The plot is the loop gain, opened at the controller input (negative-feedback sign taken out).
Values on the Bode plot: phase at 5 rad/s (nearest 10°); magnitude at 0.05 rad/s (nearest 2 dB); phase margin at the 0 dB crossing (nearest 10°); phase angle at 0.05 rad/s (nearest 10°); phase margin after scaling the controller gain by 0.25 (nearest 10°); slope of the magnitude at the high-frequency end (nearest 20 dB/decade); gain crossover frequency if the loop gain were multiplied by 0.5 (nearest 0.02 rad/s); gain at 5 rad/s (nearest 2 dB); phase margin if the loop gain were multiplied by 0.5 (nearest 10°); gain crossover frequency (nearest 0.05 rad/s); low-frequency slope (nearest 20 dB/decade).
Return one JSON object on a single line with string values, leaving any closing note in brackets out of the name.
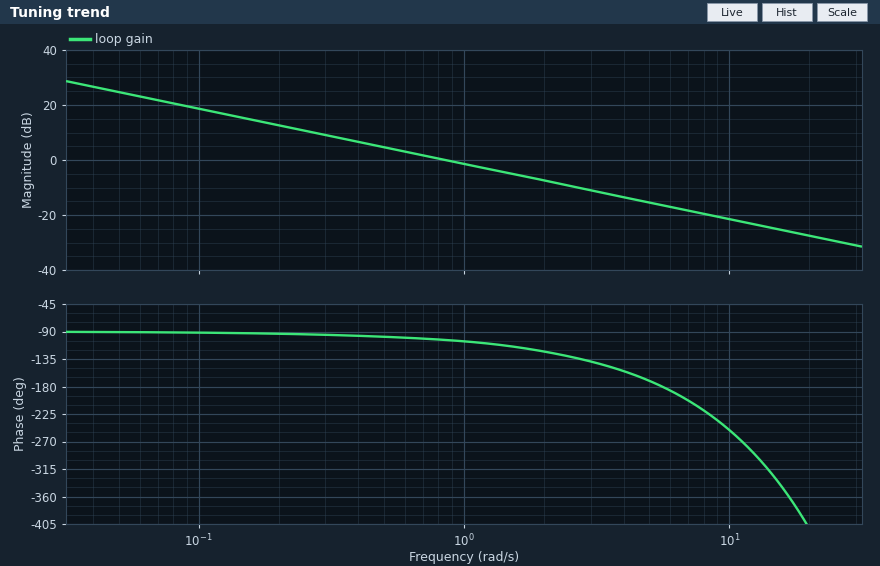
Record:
{"phase at 5 rad/s": "-170°", "magnitude at 0.05 rad/s": "24 dB", "phase margin at the 0 dB crossing": "80°", "phase angle at 0.05 rad/s": "-90°", "phase margin after scaling the controller gain by 0.25": "90°", "slope of the magnitude at the high-frequency end": "-20 dB/decade", "gain crossover frequency if the loop gain were multiplied by 0.5": "0.42 rad/s", "gain at 5 rad/s": "-16 dB", "phase margin if the loop gain were multiplied by 0.5": "80°", "gain crossover frequency": "0.85 rad/s", "low-frequency slope": "-20 dB/decade"}
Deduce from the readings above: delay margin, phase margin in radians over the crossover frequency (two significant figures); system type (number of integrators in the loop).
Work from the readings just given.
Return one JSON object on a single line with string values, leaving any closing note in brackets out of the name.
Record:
{"delay margin, phase margin in radians over the crossover frequency": "1.6 s", "system type": "1"}
